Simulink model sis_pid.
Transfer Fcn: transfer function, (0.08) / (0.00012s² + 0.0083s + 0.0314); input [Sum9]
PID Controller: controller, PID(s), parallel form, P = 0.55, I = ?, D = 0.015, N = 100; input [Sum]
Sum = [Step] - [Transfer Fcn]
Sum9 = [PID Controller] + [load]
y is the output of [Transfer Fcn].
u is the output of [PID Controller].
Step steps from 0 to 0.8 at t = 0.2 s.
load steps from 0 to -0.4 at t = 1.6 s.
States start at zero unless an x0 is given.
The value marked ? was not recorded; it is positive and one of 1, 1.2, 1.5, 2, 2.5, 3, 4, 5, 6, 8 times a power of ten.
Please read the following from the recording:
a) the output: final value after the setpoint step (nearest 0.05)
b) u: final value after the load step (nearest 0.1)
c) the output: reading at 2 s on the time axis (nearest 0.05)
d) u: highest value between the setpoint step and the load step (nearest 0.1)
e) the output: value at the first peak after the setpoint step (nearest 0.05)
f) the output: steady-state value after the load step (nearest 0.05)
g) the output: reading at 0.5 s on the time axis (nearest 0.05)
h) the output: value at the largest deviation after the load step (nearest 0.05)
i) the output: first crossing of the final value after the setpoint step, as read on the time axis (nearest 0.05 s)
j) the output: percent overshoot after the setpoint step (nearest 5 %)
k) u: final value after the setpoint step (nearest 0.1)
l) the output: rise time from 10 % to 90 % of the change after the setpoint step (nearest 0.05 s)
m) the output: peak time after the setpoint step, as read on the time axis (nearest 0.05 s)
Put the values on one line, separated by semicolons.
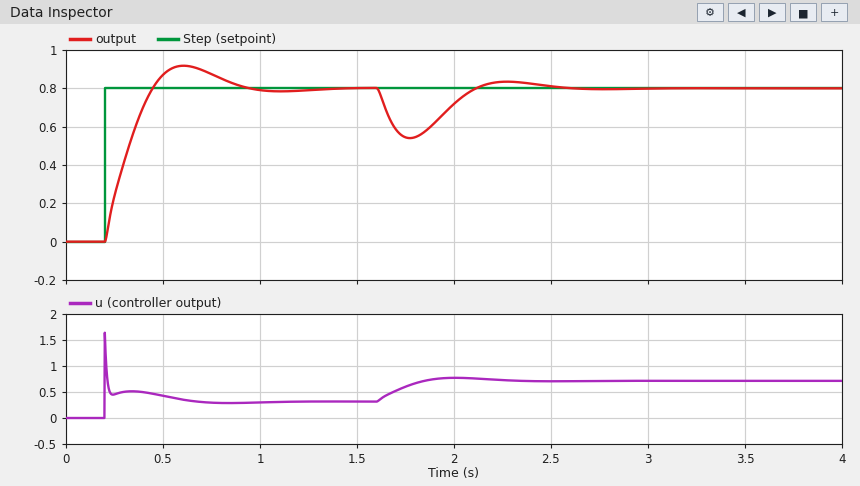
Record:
0.80; 0.7; 0.70; 1.6; 0.90; 0.80; 0.85; 0.55; 0.45 s; 15 %; 0.3; 0.20 s; 0.60 s
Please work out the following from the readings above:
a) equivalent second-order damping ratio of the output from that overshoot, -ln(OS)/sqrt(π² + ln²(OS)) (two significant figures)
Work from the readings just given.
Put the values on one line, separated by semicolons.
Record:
0.52
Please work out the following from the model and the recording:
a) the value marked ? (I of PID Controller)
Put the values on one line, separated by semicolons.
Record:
6
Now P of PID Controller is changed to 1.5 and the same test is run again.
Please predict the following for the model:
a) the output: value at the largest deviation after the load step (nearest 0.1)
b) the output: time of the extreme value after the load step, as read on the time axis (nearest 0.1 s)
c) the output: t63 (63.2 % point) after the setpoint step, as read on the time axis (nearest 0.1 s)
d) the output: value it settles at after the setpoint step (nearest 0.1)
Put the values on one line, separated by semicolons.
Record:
0.6; 1.7 s; 0.3 s; 0.8
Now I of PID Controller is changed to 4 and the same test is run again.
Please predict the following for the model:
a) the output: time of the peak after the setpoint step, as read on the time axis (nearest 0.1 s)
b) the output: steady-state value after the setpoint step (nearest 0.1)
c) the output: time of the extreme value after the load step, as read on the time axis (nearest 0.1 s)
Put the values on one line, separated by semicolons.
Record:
0.7 s; 0.8; 1.8 s
